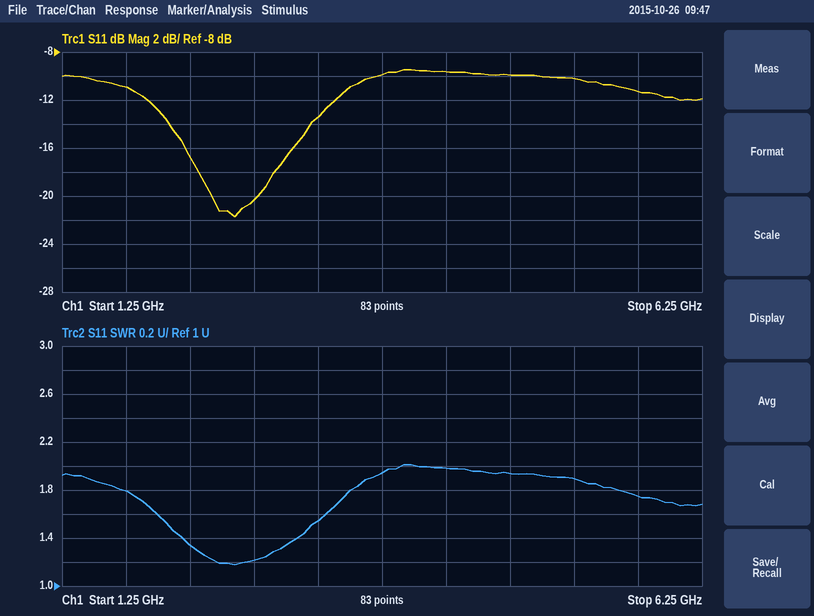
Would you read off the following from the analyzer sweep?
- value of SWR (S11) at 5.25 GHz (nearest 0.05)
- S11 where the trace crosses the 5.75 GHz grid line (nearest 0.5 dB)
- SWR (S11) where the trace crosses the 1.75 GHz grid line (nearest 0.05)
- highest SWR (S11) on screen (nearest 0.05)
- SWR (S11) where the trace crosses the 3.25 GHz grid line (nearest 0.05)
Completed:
1.90
-11.5 dB
1.80
2.00
1.55
